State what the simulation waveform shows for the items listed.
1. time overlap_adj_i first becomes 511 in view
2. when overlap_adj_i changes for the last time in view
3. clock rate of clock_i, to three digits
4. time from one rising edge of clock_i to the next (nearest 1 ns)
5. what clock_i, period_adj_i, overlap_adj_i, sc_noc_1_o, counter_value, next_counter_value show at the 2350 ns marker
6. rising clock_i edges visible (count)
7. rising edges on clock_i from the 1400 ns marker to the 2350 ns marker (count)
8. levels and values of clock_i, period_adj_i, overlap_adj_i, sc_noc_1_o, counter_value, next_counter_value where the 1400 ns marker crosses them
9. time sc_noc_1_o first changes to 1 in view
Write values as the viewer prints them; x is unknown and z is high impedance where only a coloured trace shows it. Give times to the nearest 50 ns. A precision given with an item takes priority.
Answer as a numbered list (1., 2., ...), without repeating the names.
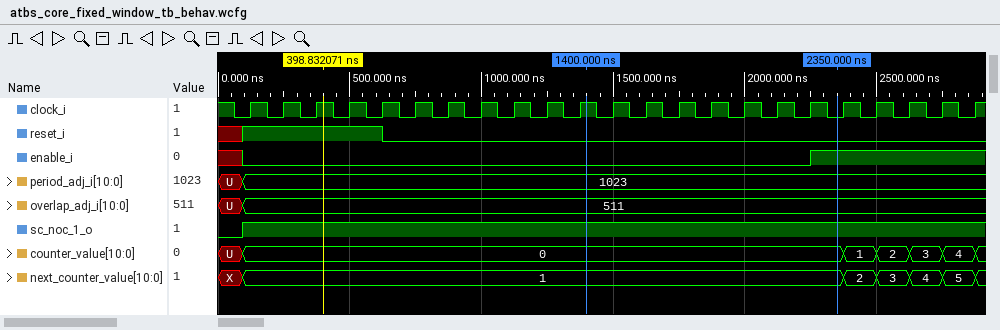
1. 100 ns
2. 100 ns
3. 8.00 MHz
4. 125 ns
5. clock_i=0, period_adj_i=1023, overlap_adj_i=511, sc_noc_1_o=1, counter_value=0, next_counter_value=1
6. 23
7. 7
8. clock_i=1, period_adj_i=1023, overlap_adj_i=511, sc_noc_1_o=1, counter_value=0, next_counter_value=1
9. 100 ns
